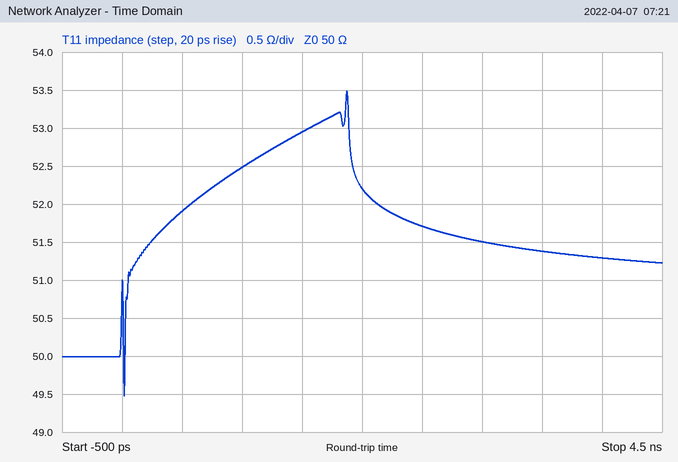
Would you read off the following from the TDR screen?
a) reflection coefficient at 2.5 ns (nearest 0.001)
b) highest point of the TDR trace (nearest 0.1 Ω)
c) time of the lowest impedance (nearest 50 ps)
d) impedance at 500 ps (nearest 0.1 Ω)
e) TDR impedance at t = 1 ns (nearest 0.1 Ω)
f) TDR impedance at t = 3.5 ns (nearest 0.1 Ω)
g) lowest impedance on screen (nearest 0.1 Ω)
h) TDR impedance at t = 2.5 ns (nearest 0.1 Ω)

+0.017
53.5 Ω
0 ps
51.9 Ω
52.5 Ω
51.4 Ω
49.5 Ω
51.7 Ω
